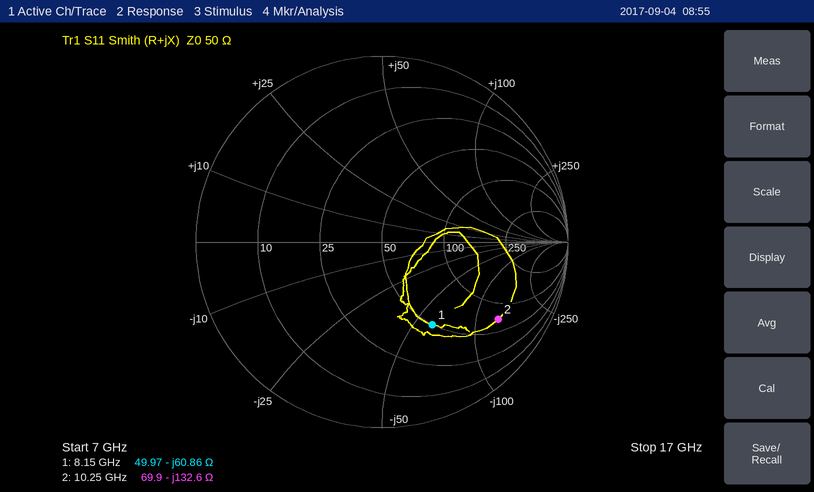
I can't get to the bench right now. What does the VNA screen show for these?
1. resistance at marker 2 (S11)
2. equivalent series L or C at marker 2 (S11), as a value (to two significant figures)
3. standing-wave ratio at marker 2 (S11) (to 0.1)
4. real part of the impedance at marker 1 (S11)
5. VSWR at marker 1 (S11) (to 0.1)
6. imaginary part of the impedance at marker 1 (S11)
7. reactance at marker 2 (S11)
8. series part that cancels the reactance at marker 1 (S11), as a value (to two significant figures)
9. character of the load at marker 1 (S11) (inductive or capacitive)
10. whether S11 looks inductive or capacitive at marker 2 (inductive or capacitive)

69.9 Ω
120 fF
7.0
49.97 Ω
3.2
-60.86 Ω
-132.6 Ω
1.2 nH
capacitive
capacitive
